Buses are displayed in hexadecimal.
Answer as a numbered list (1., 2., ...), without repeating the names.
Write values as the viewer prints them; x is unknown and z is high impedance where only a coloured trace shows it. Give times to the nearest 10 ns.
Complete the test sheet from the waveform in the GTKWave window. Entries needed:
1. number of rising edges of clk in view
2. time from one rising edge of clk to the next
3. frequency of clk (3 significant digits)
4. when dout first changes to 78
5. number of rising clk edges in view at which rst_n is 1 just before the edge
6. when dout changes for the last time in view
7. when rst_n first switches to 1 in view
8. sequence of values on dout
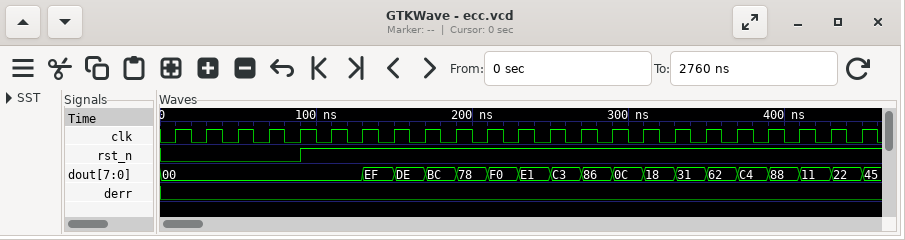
1. 23
2. 20 ns
3. 50.0 MHz
4. 190 ns
5. 18
6. 450 ns
7. 90 ns
8. 00, EF, DE, BC, 78, F0, E1, C3, 86, 0C, 18, 31, 62, C4, 88, 11, 22, 45
